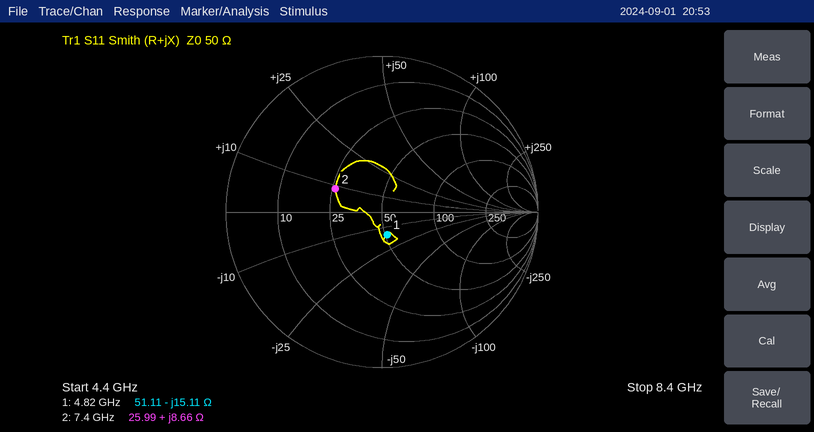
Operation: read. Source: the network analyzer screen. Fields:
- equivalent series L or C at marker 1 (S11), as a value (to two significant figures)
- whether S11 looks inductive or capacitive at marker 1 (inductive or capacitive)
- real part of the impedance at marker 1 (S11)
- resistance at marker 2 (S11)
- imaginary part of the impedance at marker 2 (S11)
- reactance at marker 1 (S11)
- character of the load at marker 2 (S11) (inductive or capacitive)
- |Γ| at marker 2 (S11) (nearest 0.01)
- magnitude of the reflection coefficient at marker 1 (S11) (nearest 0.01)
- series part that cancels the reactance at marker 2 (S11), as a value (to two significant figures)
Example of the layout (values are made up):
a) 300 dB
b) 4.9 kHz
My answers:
a) 2.2 pF
b) capacitive
c) 51.11 Ω
d) 25.99 Ω
e) +8.66 Ω
f) -15.11 Ω
g) inductive
h) 0.33
i) 0.15
j) 2.5 pF
